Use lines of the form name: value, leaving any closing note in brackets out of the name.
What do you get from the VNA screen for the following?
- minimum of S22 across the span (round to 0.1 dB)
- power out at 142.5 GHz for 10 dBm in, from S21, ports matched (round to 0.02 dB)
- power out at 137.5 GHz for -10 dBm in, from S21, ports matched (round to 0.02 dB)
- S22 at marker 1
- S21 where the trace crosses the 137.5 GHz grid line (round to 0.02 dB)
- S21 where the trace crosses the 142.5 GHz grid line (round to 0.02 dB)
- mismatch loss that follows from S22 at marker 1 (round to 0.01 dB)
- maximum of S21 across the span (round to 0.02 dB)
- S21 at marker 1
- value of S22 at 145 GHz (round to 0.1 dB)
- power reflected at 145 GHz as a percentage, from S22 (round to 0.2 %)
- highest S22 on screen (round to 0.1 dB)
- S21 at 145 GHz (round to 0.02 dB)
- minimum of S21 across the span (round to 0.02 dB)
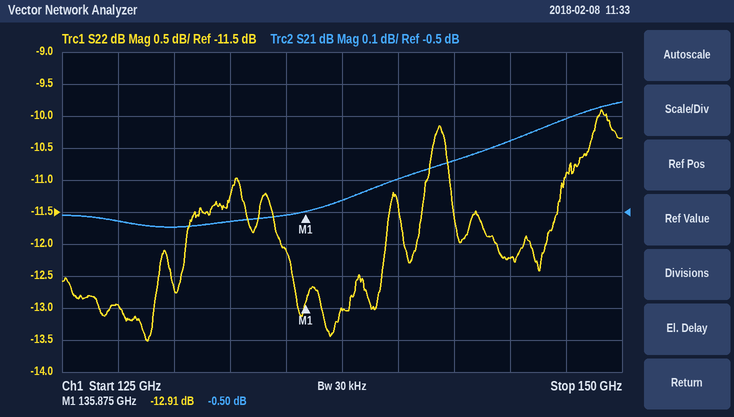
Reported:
minimum of S22 across the span: -13.5 dB
power out at 142.5 GHz for 10 dBm in, from S21, ports matched: 9.66 dBm
power out at 137.5 GHz for -10 dBm in, from S21, ports matched: -10.46 dBm
S22 at marker 1: -12.91 dB
S21 where the trace crosses the 137.5 GHz grid line: -0.46 dB
S21 where the trace crosses the 142.5 GHz grid line: -0.34 dB
mismatch loss that follows from S22 at marker 1: 0.23 dB
maximum of S21 across the span: -0.16 dB
S21 at marker 1: -0.50 dB
value of S22 at 145 GHz: -12.2 dB
power reflected at 145 GHz as a percentage, from S22: 6.0 %
highest S22 on screen: -9.9 dB
S21 at 145 GHz: -0.28 dB
minimum of S21 across the span: -0.54 dB
